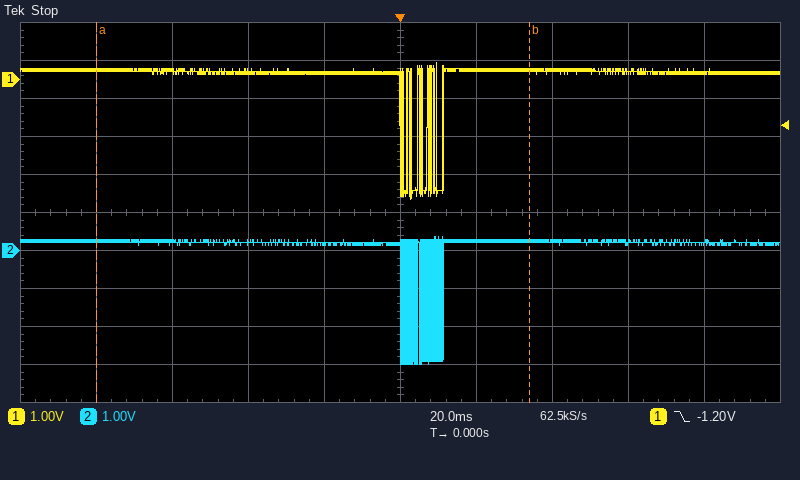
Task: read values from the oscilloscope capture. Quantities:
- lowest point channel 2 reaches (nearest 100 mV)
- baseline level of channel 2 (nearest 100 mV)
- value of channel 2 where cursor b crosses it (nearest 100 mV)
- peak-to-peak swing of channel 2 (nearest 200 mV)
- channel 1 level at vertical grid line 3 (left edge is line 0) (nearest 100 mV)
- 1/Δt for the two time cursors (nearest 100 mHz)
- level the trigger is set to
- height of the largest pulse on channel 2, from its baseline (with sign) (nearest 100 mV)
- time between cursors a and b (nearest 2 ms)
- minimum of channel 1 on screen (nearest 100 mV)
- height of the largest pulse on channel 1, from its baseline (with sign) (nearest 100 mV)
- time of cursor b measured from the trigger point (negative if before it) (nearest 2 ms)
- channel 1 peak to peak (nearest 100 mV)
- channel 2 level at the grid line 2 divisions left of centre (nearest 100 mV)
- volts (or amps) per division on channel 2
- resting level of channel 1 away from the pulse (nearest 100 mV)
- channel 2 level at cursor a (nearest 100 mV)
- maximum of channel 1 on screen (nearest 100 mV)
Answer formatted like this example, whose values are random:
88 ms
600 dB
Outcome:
-3.0 V
200 mV
200 mV
3.4 V
200 mV
8.8 Hz
-1.20 V
-3.2 V
114 ms
-3.2 V
-3.4 V
+34 ms
3.6 V
200 mV
1 V
200 mV
200 mV
400 mV
